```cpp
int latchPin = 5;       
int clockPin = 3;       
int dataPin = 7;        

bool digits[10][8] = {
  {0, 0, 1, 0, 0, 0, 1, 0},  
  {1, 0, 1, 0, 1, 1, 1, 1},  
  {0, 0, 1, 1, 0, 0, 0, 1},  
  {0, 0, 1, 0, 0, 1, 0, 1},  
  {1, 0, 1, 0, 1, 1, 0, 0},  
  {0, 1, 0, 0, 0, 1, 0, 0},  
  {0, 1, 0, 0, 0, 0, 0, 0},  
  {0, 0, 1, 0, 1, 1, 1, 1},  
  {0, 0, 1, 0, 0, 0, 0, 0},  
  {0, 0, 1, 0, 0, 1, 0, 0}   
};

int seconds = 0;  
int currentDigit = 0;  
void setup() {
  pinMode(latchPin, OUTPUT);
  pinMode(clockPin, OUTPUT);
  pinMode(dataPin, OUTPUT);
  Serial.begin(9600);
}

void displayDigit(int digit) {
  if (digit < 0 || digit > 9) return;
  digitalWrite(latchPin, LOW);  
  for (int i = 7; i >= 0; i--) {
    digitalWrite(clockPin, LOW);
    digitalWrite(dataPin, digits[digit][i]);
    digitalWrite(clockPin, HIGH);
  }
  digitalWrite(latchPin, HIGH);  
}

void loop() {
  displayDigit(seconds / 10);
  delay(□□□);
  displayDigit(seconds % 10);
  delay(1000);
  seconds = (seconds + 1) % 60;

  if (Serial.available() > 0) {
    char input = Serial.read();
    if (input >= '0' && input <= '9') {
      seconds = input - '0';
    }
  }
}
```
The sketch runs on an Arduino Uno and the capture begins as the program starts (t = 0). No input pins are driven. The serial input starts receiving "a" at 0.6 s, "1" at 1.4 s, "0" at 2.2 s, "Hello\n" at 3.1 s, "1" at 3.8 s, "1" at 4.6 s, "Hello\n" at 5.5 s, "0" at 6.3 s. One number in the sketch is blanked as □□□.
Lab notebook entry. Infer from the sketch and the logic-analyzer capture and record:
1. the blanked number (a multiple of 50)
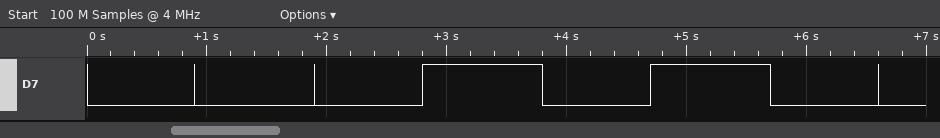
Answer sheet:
900
